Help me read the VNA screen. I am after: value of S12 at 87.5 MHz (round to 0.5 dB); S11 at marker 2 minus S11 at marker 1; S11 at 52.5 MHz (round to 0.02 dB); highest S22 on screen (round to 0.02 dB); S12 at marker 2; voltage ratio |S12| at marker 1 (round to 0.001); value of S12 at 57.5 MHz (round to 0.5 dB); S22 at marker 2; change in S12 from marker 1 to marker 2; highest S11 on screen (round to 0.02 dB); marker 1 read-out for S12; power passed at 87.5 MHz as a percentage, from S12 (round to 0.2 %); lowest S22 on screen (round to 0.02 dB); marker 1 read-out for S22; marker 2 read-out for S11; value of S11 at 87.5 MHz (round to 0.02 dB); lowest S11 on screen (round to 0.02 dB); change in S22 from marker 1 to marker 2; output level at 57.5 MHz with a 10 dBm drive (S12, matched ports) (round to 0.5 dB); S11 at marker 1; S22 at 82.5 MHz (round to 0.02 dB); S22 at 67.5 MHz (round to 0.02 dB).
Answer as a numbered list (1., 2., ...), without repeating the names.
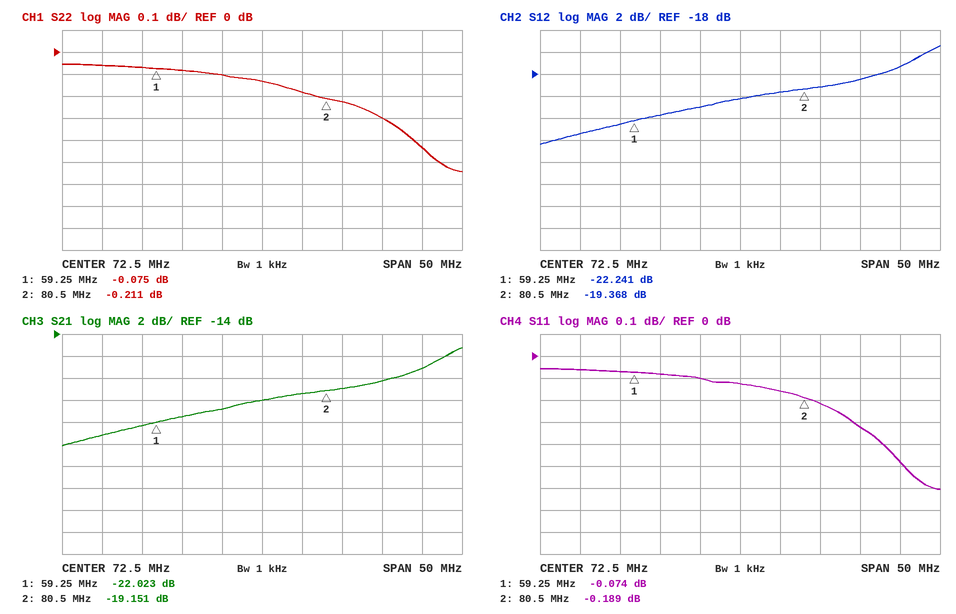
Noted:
1. -18.5 dB
2. -0.115 dB
3. -0.06 dB
4. -0.06 dB
5. -19.368 dB
6. 0.077
7. -22.5 dB
8. -0.211 dB
9. 2.873 dB
10. -0.06 dB
11. -22.241 dB
12. 1.4 %
13. -0.54 dB
14. -0.075 dB
15. -0.189 dB
16. -0.32 dB
17. -0.60 dB
18. -0.136 dB
19. -12.5 dBm
20. -0.074 dB
21. -0.22 dB
22. -0.10 dB
